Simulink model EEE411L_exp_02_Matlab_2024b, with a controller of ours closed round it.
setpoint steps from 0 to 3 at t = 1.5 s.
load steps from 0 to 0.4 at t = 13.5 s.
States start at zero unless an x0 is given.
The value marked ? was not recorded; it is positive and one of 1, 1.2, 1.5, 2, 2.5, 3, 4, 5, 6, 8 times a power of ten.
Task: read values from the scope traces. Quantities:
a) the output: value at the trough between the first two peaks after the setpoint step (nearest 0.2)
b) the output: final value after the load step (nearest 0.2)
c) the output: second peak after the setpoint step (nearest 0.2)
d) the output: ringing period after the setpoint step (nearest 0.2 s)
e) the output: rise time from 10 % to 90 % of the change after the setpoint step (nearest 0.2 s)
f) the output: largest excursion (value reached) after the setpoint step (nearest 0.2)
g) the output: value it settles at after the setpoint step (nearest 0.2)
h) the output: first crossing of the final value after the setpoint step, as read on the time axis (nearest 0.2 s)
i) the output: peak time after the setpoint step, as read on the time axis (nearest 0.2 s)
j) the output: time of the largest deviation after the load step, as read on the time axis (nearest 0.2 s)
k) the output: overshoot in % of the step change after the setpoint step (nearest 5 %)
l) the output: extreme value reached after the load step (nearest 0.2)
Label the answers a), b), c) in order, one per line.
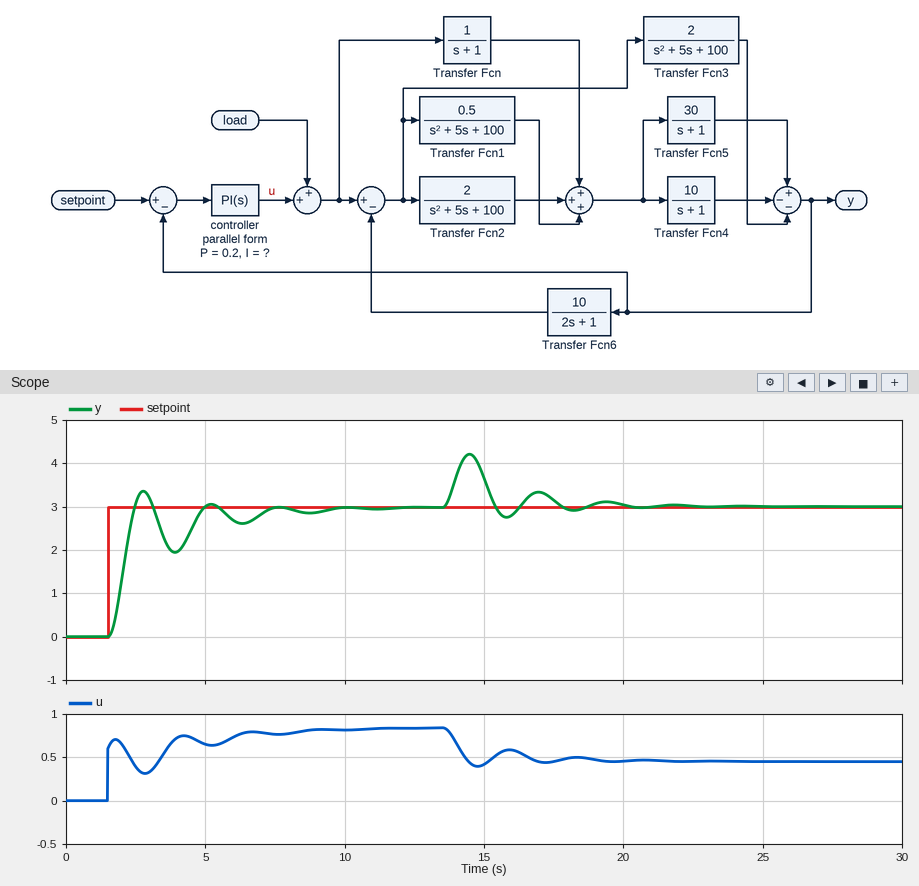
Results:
a) 2.0
b) 3.0
c) 3.0
d) 2.4 s
e) 0.6 s
f) 3.4
g) 3.0
h) 2.4 s
i) 2.8 s
j) 14.4 s
k) 10 %
l) 4.2
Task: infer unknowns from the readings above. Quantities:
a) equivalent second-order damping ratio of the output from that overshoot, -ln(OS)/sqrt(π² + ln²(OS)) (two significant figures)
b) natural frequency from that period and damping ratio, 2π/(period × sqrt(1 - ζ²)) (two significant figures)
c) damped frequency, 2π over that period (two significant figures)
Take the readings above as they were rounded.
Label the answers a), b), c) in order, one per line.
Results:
a) 0.59
b) 3.2 rad/s
c) 2.6 rad/s
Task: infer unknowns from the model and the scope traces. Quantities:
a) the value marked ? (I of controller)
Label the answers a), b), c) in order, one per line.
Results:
a) 0.25
